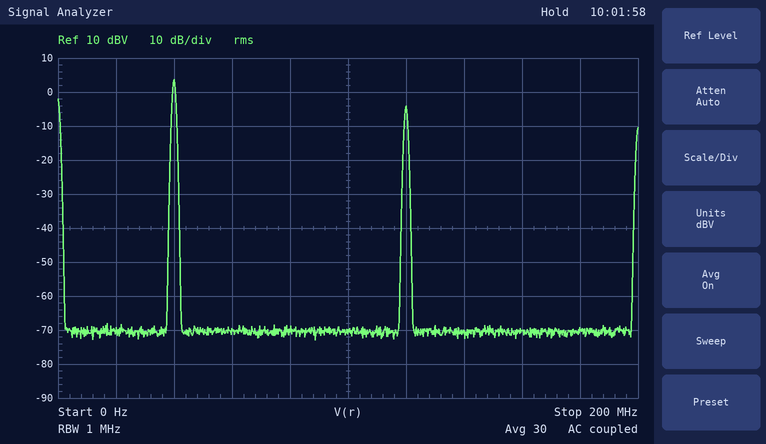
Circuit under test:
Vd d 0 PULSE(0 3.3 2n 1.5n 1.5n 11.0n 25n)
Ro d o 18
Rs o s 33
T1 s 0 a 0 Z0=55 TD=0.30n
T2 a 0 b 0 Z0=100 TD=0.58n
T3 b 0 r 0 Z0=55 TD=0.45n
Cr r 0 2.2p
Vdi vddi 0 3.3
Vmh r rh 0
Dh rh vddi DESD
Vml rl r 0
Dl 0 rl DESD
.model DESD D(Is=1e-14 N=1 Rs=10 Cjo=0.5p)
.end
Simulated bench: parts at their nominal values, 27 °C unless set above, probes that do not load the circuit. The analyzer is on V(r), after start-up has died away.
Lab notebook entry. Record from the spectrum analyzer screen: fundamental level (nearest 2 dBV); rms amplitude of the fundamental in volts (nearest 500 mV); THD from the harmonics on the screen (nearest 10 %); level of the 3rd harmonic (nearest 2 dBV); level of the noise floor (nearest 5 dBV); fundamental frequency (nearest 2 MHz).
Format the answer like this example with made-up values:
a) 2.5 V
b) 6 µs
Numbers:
a) 4 dBV
b) 1.5 V
c) 40 %
d) -4 dBV
e) -70 dBV
f) 40 MHz
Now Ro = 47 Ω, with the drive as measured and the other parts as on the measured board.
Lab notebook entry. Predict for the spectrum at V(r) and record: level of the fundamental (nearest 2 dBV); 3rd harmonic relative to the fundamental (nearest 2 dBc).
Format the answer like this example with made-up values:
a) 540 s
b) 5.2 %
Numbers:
a) 4 dBV
b) -10 dBc
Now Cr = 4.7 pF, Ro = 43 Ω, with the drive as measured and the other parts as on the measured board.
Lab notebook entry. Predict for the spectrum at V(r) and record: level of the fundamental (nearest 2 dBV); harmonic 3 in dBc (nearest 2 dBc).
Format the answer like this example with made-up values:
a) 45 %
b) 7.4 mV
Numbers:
a) 4 dBV
b) -10 dBc
